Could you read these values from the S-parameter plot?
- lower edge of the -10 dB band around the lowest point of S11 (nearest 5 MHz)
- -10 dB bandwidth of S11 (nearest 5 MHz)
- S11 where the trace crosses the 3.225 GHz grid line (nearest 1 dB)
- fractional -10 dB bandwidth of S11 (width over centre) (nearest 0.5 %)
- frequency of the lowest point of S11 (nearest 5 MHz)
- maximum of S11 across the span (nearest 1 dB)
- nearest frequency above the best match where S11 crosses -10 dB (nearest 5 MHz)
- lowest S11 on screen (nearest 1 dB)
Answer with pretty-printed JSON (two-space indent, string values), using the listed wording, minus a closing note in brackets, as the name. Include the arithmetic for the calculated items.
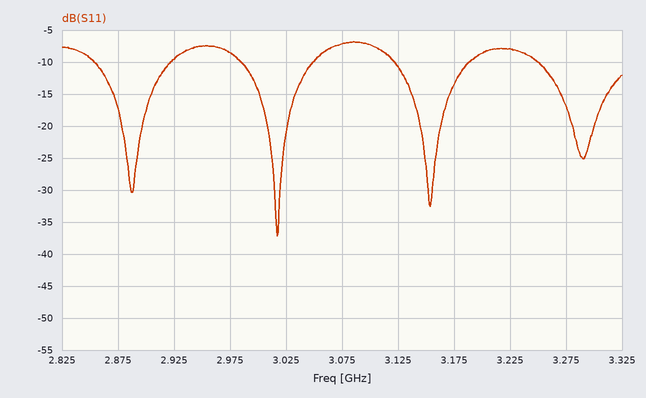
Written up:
{
  "lower edge of the -10 dB band around the lowest point of S11": "2.985 GHz",
  "-10 dB bandwidth of S11": "3.050 GHz − 2.985 GHz = 65 MHz",
  "S11 where the trace crosses the 3.225 GHz grid line": "-8 dB",
  "fractional -10 dB bandwidth of S11 (width over centre)": "65 MHz / 3.0175 GHz ≈ 2.15 %, so 2.0 % to the nearest 0.5 %",
  "frequency of the lowest point of S11": "3.015 GHz",
  "maximum of S11 across the span": "-7 dB",
  "nearest frequency above the best match where S11 crosses -10 dB": "3.050 GHz",
  "lowest S11 on screen": "-37 dB"
}
